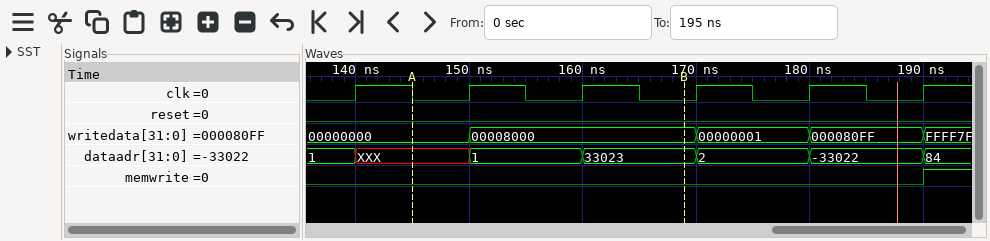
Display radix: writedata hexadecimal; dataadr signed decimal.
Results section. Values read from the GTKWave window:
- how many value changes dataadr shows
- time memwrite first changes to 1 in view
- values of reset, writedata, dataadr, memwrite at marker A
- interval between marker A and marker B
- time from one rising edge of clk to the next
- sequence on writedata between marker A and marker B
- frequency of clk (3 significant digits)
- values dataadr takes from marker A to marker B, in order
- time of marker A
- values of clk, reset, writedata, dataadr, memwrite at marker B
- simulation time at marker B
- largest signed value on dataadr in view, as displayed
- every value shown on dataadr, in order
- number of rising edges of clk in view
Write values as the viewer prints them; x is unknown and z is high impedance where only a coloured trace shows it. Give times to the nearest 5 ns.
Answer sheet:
6
190 ns
reset=0, writedata=00000000, dataadr=XXX, memwrite=0
25 ns
10 ns
00000000, 00008000
100 MHz
XXX, 1, 33023
145 ns
clk=0, reset=0, writedata=00008000, dataadr=33023, memwrite=0
170 ns
33023
1, XXX, 1, 33023, 2, -33022, 84
6
